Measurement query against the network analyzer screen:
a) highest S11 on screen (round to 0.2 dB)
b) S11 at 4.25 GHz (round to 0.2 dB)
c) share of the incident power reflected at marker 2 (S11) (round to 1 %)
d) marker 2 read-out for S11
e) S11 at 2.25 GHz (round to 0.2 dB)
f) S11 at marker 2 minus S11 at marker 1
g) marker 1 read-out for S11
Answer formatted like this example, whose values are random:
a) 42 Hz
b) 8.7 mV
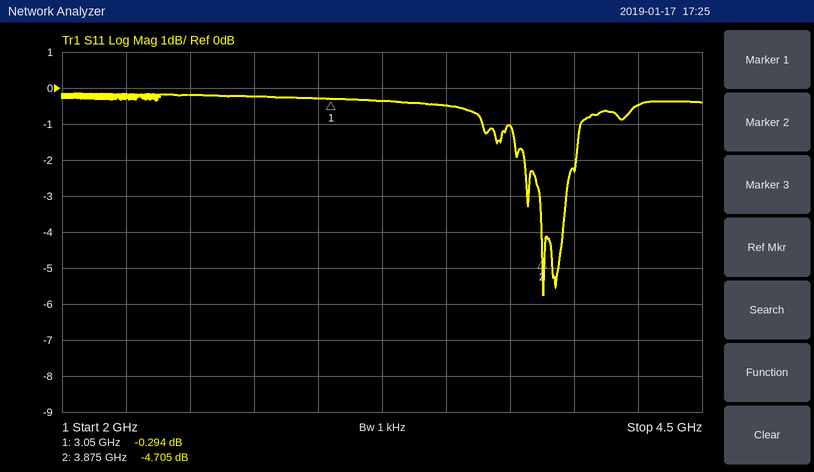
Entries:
a) -0.2 dB
b) -0.4 dB
c) 34 %
d) -4.705 dB
e) -0.2 dB
f) -4.411 dB
g) -0.294 dB
